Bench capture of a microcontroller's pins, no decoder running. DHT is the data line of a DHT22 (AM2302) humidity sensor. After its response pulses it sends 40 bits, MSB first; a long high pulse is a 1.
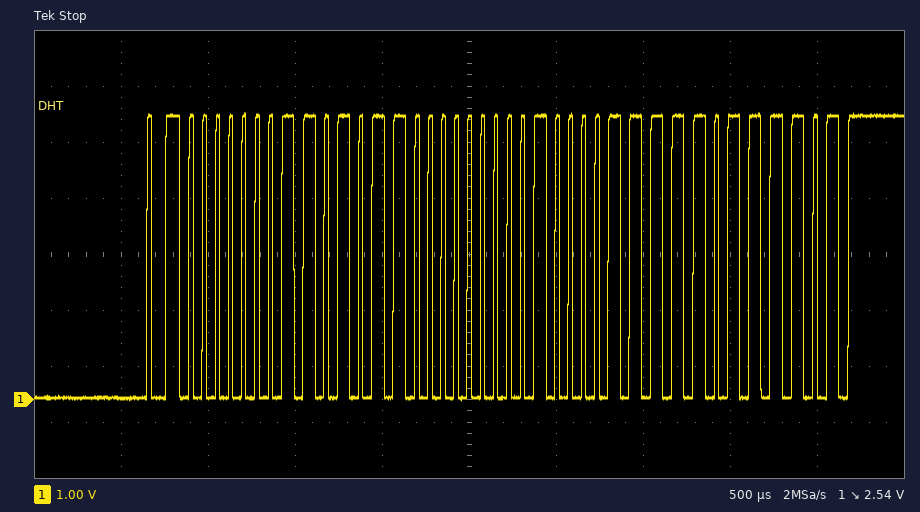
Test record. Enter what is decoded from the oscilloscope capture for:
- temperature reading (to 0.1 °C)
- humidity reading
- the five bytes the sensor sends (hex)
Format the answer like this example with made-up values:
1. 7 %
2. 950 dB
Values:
1. 27.1 °C
2. 42.8 %
3. 01 AC 01 0F BD
